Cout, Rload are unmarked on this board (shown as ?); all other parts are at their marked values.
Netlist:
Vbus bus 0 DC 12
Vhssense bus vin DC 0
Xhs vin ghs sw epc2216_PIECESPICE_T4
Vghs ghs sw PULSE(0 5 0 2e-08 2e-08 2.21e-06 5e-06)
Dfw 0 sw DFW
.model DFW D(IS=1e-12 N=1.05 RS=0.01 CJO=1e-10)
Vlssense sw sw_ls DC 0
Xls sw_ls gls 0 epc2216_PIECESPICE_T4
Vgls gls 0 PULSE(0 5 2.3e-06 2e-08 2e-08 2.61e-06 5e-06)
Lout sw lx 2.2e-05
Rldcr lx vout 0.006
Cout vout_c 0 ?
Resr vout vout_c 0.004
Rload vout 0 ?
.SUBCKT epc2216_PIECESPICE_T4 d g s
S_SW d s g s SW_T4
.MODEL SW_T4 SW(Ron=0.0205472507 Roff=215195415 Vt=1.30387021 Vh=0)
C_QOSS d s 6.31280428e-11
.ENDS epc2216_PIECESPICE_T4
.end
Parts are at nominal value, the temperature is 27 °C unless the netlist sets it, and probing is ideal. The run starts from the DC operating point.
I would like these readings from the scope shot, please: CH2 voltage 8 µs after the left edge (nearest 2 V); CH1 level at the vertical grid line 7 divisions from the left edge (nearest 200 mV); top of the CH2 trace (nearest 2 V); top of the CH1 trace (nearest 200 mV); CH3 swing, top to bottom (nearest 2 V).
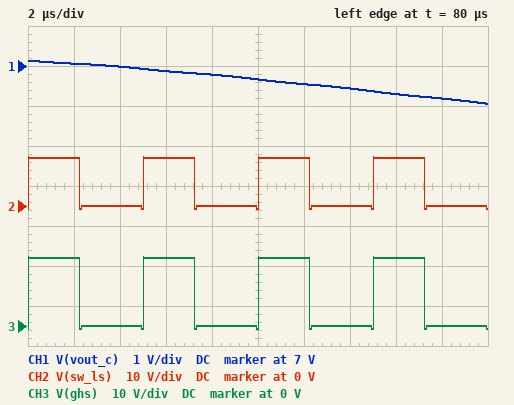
0 V
6.4 V
12 V
7.2 V
18 V
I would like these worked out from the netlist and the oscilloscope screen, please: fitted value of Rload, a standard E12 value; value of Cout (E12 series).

1.8 Ω
22 µF
